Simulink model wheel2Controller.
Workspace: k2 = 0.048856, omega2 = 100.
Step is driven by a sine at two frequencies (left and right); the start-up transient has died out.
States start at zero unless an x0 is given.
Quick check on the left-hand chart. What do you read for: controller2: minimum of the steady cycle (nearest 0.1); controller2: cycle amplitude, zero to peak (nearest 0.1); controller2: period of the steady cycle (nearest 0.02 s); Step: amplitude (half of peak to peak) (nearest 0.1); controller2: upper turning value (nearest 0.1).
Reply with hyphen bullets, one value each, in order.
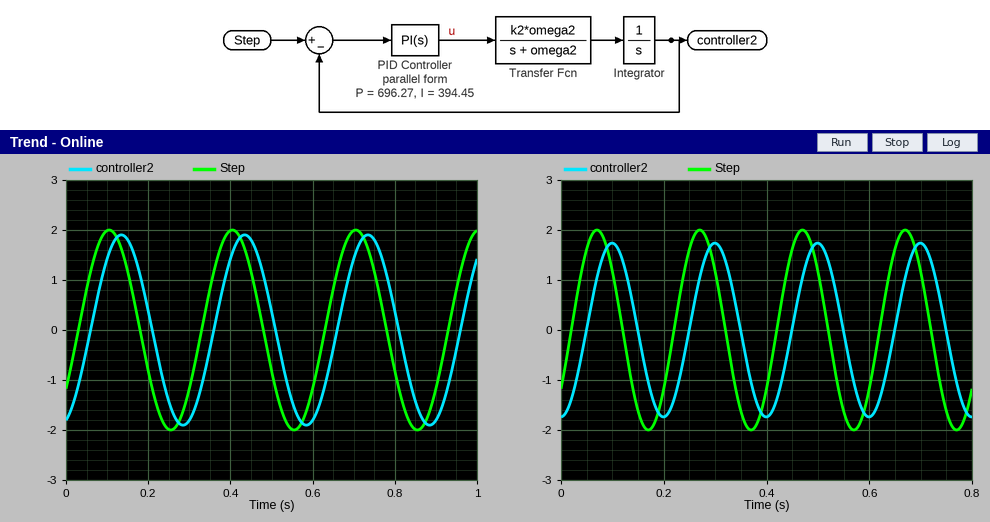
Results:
- -1.9
- 1.9
- 0.30 s
- 2.0
- 1.9
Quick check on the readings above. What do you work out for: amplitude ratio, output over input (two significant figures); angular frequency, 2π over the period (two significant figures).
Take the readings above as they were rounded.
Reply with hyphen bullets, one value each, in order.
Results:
- 0.95
- 21 rad/s
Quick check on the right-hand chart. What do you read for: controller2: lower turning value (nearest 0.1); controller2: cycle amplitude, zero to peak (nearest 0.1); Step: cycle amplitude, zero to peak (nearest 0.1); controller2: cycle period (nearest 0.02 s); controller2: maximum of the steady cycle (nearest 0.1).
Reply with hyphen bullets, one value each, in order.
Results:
- -1.7
- 1.7
- 2.0
- 0.20 s
- 1.7
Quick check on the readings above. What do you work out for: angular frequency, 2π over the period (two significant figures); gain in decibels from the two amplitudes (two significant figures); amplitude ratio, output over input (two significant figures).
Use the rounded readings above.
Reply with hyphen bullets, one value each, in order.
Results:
- 31 rad/s
- -1.4 dB
- 0.85
